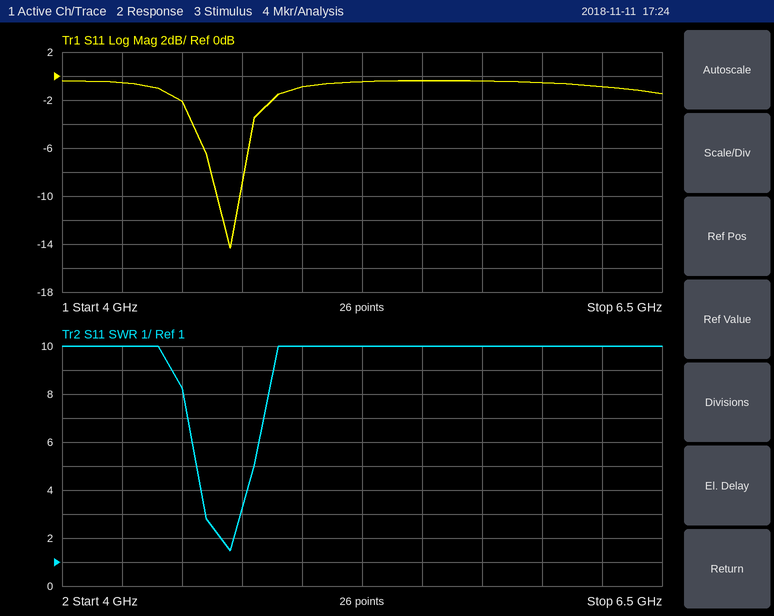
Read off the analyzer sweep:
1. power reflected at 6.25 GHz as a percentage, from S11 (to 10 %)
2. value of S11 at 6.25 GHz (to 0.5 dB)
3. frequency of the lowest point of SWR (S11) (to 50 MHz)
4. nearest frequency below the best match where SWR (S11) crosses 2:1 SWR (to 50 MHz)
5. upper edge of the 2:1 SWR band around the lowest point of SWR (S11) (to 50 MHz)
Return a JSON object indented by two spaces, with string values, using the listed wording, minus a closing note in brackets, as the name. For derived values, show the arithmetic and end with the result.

{
  "power reflected at 6.25 GHz as a percentage, from S11": "10^(-1/10) ≈ 79.4 %, so 80 % to the nearest 10 %",
  "value of S11 at 6.25 GHz": "-1.0 dB",
  "frequency of the lowest point of SWR (S11)": "4.70 GHz",
  "nearest frequency below the best match where SWR (S11) crosses 2:1 SWR": "4.65 GHz",
  "upper edge of the 2:1 SWR band around the lowest point of SWR (S11)": "4.70 GHz"
}
